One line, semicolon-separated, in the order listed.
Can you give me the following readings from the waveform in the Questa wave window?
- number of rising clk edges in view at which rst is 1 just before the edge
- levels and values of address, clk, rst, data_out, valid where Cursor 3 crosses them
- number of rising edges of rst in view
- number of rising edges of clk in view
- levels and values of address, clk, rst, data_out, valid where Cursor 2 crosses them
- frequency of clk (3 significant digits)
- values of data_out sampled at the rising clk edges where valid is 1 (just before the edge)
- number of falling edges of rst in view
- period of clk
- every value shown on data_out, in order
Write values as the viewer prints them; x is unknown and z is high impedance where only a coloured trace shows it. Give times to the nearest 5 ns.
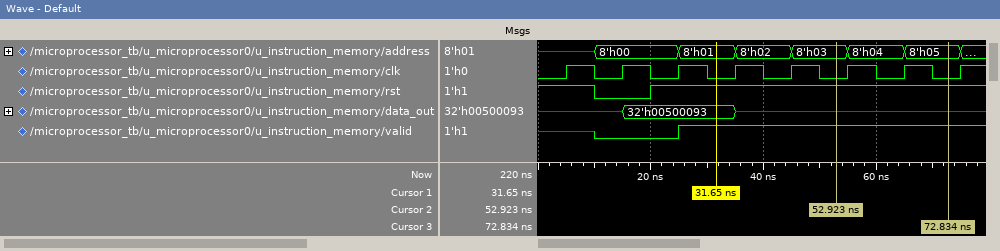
7; address=8'h05, clk=0, rst=1, data_out=x, valid=1; 1; 8; address=8'h03, clk=0, rst=1, data_out=x, valid=1; 100 MHz; 32'h00500093, x, x, x, x; 1; 10 ns; x, 32'h00500093, x
